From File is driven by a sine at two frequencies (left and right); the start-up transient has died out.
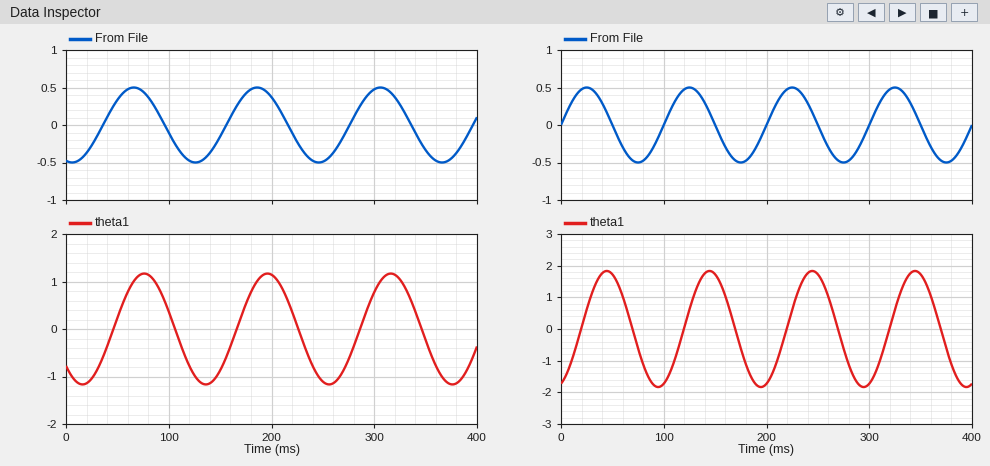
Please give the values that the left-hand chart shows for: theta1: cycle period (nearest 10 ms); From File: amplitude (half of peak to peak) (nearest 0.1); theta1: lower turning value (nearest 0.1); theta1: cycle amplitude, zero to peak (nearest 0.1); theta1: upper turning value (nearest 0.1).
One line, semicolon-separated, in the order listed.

120 ms; 0.5; -1.2; 1.2; 1.2
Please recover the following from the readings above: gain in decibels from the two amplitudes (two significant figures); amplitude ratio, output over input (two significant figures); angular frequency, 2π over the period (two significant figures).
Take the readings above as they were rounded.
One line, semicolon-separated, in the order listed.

7.6 dB; 2.4; 0.052 rad/ms
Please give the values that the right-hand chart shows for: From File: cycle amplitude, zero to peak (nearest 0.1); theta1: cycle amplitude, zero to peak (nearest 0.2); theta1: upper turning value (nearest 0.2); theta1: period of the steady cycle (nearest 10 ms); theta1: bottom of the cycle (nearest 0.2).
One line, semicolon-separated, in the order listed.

0.5; 1.8; 1.8; 100 ms; -1.8
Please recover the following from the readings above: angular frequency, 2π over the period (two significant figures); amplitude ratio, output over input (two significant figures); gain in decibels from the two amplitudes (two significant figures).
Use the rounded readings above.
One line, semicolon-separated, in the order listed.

0.063 rad/ms; 3.6; 11 dB
